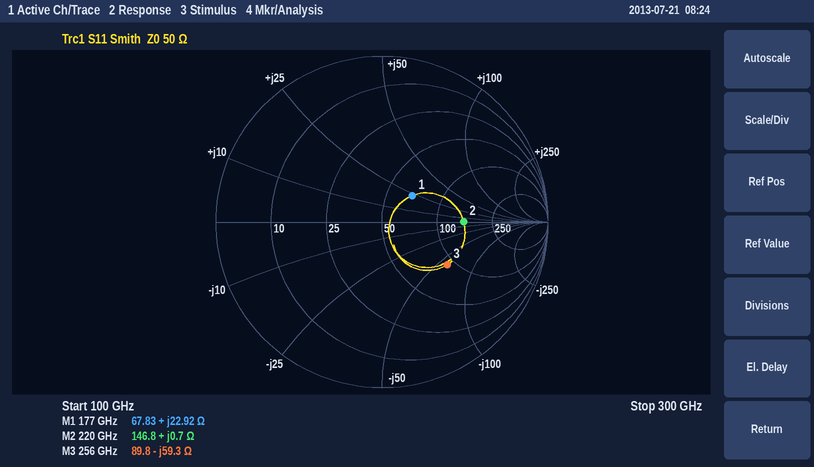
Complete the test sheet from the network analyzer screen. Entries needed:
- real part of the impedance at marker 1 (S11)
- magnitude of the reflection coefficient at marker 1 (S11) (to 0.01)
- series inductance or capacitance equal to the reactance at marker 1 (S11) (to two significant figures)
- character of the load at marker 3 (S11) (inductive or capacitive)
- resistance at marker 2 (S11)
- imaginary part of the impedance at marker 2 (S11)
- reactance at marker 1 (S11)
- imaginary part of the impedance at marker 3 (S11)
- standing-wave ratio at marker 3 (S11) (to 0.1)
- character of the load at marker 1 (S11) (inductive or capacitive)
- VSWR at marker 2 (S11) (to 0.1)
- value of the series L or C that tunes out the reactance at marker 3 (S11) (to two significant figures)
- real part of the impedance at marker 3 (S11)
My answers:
67.83 Ω
0.24
21 pH
capacitive
146.8 Ω
+0.7 Ω
+22.92 Ω
-59.3 Ω
2.8
inductive
2.9
37 pH
89.8 Ω
